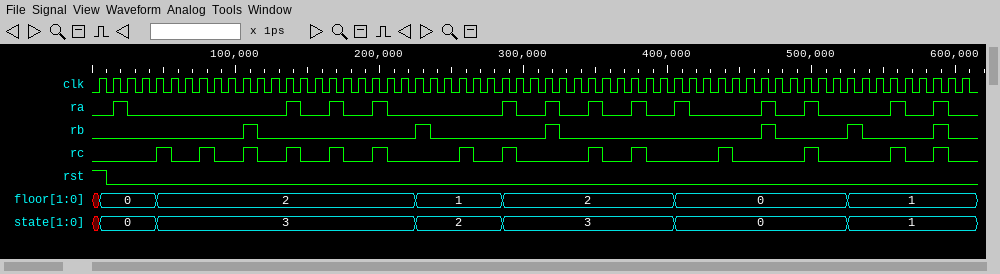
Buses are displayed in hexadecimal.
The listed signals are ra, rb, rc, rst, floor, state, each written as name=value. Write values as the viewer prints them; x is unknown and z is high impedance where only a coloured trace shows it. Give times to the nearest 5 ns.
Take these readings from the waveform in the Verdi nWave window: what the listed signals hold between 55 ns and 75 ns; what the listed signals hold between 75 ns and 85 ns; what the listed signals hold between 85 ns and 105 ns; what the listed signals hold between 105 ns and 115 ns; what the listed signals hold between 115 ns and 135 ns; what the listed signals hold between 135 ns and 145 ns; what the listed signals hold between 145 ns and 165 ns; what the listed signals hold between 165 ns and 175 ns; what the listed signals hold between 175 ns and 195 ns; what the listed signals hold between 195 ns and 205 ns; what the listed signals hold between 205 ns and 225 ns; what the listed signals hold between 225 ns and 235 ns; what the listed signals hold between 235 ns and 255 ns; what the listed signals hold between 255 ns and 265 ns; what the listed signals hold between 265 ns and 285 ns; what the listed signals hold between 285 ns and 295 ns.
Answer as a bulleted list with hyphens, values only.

- ra=0, rb=0, rc=0, rst=0, floor=2, state=3
- ra=0, rb=0, rc=1, rst=0, floor=2, state=3
- ra=0, rb=0, rc=0, rst=0, floor=2, state=3
- ra=0, rb=1, rc=1, rst=0, floor=2, state=3
- ra=0, rb=0, rc=0, rst=0, floor=2, state=3
- ra=1, rb=0, rc=1, rst=0, floor=2, state=3
- ra=0, rb=0, rc=0, rst=0, floor=2, state=3
- ra=1, rb=0, rc=1, rst=0, floor=2, state=3
- ra=0, rb=0, rc=0, rst=0, floor=2, state=3
- ra=1, rb=0, rc=1, rst=0, floor=2, state=3
- ra=0, rb=0, rc=0, rst=0, floor=2, state=3
- ra=0, rb=1, rc=0, rst=0, floor=1, state=2
- ra=0, rb=0, rc=0, rst=0, floor=1, state=2
- ra=0, rb=0, rc=1, rst=0, floor=1, state=2
- ra=0, rb=0, rc=0, rst=0, floor=1, state=2
- ra=1, rb=0, rc=1, rst=0, floor=2, state=3
